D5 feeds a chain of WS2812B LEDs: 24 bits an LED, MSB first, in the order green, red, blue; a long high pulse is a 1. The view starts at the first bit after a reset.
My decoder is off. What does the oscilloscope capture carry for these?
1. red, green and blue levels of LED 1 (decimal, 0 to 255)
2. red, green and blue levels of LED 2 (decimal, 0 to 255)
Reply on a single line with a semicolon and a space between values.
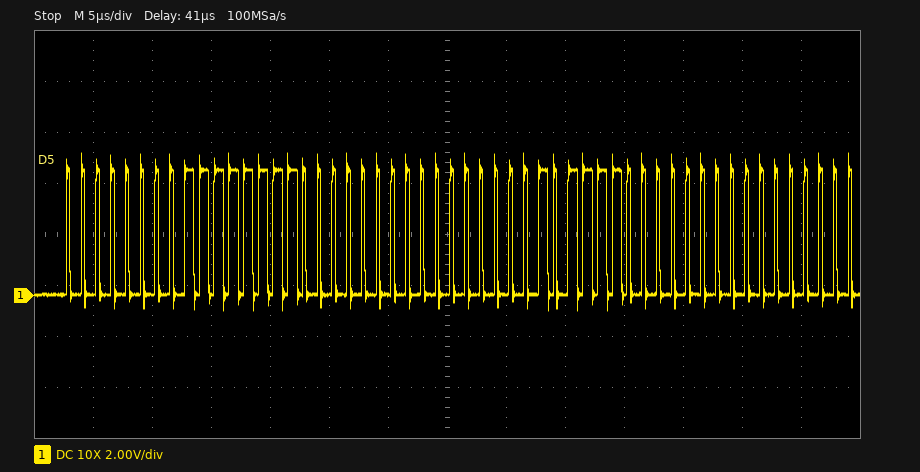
255, 0, 0; 188, 0, 0
